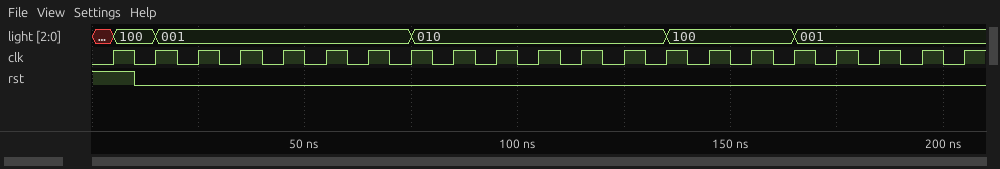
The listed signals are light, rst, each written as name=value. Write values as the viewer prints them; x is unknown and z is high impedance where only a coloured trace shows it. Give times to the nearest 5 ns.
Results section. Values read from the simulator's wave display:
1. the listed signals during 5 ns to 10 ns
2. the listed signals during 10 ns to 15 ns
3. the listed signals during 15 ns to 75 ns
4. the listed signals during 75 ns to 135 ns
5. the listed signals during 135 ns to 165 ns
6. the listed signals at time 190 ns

light=100, rst=1
light=100, rst=0
light=001, rst=0
light=010, rst=0
light=100, rst=0
light=001, rst=0
